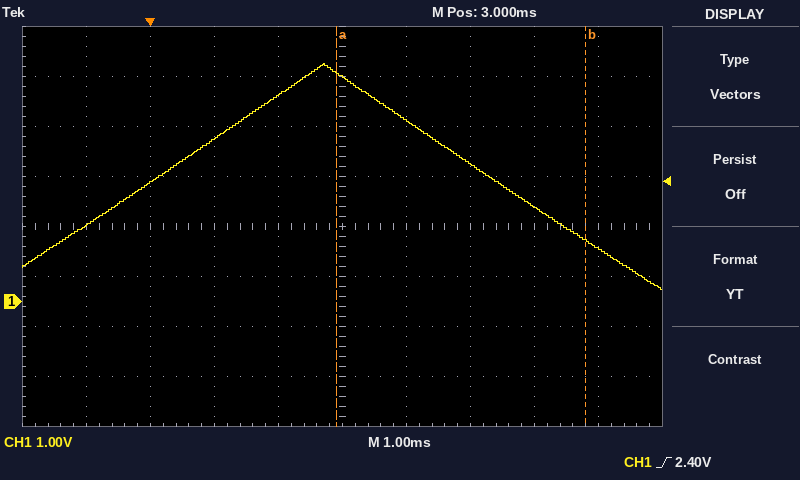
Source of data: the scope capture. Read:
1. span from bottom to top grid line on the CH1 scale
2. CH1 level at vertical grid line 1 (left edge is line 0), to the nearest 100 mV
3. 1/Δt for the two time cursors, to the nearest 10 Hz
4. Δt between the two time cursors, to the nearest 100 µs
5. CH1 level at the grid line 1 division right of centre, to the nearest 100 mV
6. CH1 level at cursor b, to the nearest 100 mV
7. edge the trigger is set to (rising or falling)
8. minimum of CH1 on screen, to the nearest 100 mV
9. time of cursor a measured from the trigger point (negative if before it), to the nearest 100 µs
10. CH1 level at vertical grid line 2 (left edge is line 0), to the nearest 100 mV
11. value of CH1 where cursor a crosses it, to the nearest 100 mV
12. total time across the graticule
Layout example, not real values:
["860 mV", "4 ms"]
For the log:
["8 V", "1.5 V", "260 Hz", "3.9 ms", "3.6 V", "1.2 V", "rising", "200 mV", "+2.9 ms", "2.4 V", "4.6 V", "10 ms"]
